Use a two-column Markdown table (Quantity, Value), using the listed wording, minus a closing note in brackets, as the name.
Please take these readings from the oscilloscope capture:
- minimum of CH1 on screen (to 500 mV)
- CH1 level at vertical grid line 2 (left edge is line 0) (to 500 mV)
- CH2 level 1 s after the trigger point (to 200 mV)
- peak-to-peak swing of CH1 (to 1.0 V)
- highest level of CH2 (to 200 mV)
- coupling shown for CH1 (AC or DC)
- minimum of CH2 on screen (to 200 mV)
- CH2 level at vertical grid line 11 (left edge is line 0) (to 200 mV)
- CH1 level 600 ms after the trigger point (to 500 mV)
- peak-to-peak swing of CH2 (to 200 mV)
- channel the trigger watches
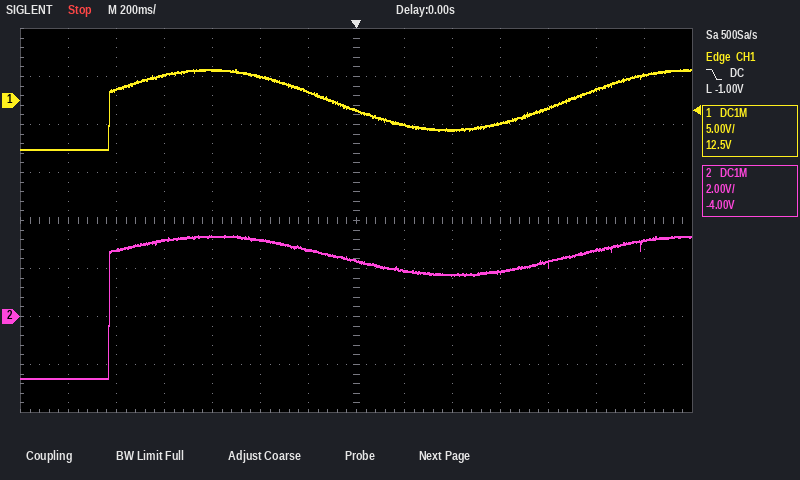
| Quantity | Value |
|---|---|
| minimum of CH1 on screen | -5.0 V |
| CH1 level at vertical grid line 2 (left edge is line 0) | 1.0 V |
| CH2 level 1 s after the trigger point | 2.8 V |
| peak-to-peak swing of CH1 | 8.0 V |
| highest level of CH2 | 3.4 V |
| coupling shown for CH1 | DC |
| minimum of CH2 on screen | -2.6 V |
| CH2 level at vertical grid line 11 (left edge is line 0) | 2.2 V |
| CH1 level 600 ms after the trigger point | -2.5 V |
| peak-to-peak swing of CH2 | 6.0 V |
| channel the trigger watches | CH1 |
